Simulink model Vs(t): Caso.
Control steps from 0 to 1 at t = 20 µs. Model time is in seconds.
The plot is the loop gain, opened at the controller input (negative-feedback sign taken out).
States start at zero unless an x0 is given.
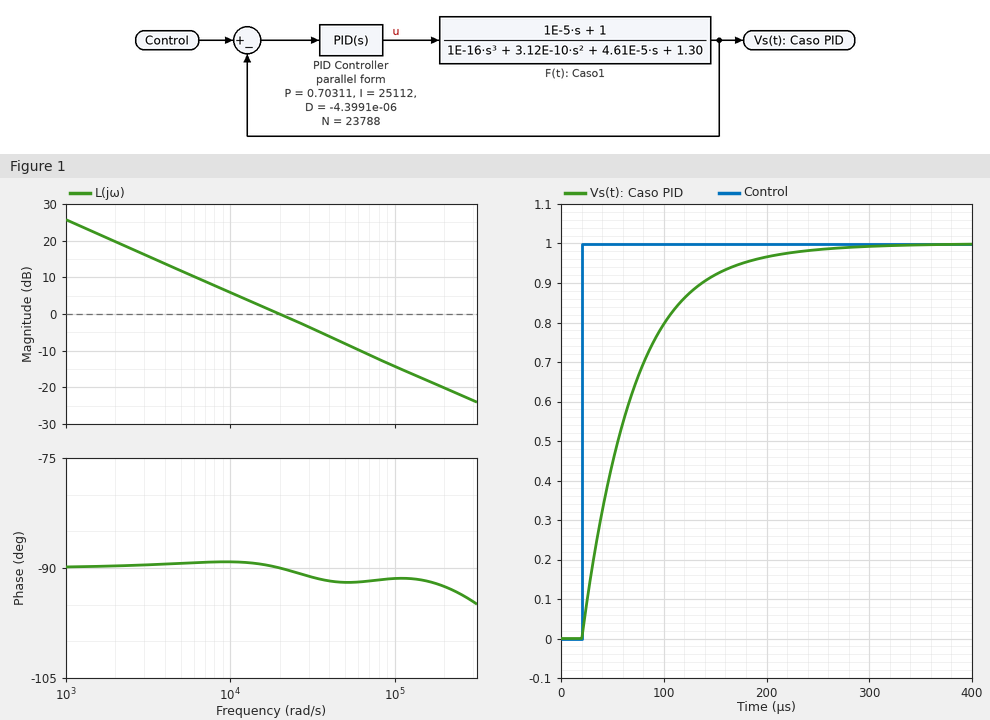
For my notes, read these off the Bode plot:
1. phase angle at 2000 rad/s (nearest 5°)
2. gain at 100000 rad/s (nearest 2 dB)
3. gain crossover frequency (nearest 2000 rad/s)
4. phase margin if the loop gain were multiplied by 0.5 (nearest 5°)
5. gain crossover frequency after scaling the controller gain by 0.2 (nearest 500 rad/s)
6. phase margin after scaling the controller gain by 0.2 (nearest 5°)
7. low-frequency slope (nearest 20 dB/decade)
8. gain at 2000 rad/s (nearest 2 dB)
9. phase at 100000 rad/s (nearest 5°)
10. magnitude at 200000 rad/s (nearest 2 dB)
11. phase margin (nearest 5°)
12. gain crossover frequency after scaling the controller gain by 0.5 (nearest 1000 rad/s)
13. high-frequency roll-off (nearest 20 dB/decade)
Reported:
-90°
-14 dB
20000 rad/s
90°
4000 rad/s
90°
-20 dB/decade
20 dB
-90°
-20 dB
90°
10000 rad/s
-20 dB/decade
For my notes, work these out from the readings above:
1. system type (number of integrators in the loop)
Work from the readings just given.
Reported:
1
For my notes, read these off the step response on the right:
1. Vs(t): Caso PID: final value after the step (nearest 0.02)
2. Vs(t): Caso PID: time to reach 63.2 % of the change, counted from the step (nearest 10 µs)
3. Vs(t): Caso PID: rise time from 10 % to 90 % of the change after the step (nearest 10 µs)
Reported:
1.00
50 µs
110 µs
